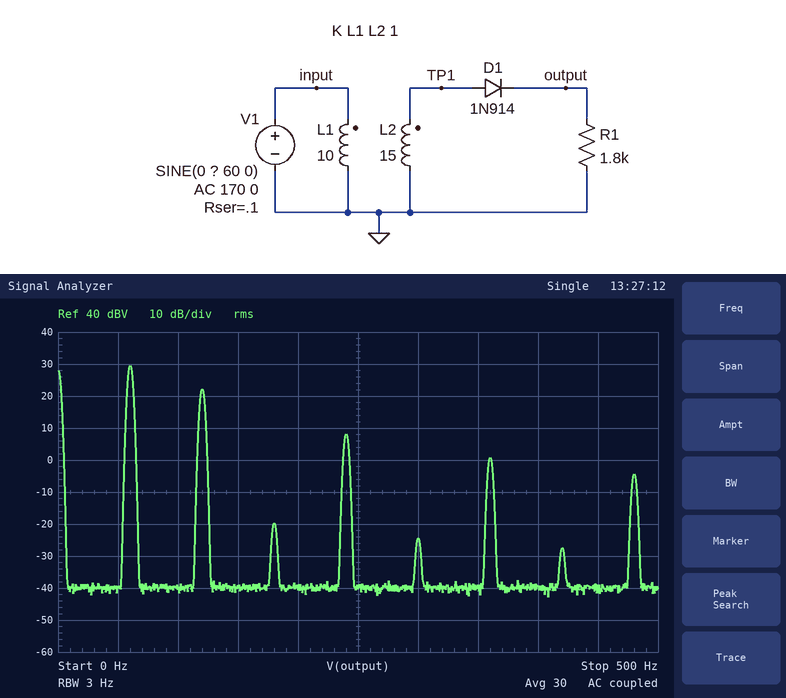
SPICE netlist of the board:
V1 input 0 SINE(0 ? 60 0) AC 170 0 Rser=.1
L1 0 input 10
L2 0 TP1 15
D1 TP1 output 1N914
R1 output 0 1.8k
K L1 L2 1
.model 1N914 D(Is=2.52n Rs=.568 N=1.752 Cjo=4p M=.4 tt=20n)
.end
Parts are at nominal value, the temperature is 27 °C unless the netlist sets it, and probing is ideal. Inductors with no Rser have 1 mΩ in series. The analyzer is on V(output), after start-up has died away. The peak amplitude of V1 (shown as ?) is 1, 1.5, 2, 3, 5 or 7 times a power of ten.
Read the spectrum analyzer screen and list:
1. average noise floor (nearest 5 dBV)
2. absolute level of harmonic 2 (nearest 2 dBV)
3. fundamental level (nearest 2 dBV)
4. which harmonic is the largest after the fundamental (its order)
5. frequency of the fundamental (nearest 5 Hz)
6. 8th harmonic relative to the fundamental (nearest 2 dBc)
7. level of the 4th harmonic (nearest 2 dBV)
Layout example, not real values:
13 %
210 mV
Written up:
-40 dBV
22 dBV
30 dBV
2
60 Hz
-34 dBc
8 dBV
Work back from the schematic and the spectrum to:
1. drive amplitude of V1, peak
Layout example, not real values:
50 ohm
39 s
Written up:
70 V
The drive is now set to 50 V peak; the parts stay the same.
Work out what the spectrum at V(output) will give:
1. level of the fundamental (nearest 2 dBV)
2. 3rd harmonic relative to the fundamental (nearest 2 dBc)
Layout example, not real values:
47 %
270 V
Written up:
26 dBV
-46 dBc
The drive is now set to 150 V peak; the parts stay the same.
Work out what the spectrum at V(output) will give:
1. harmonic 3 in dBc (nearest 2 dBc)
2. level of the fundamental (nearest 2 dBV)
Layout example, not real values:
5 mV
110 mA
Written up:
-56 dBc
36 dBV
